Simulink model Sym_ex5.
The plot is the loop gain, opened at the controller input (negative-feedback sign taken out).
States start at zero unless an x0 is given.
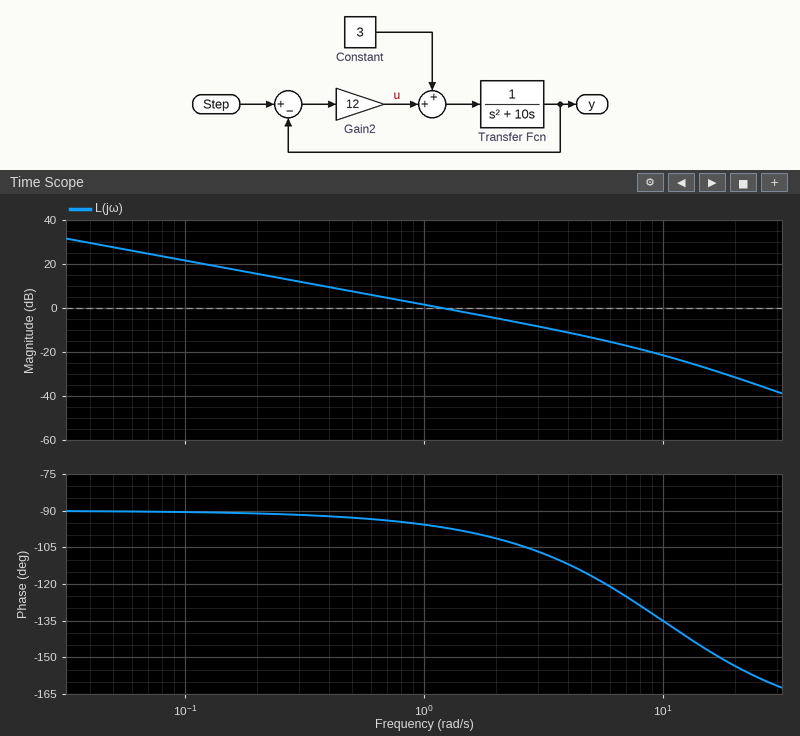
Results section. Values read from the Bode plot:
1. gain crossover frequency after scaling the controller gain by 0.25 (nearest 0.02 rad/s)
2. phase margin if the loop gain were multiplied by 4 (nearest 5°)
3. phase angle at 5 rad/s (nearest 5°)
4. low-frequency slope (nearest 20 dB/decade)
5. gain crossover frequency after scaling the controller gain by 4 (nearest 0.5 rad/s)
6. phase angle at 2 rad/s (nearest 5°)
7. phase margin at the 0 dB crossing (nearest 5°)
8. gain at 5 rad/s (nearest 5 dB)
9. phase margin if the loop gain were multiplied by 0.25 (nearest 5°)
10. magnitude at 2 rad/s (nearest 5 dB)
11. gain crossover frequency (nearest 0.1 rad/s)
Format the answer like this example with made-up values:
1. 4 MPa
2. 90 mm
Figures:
1. 0.30 rad/s
2. 65°
3. -115°
4. -20 dB/decade
5. 4.5 rad/s
6. -100°
7. 85°
8. -15 dB
9. 90°
10. -5 dB
11. 1.2 rad/s
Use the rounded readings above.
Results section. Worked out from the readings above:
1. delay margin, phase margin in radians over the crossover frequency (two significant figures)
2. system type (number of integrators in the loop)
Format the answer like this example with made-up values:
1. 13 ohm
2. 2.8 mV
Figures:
1. 1.2 s
2. 1
